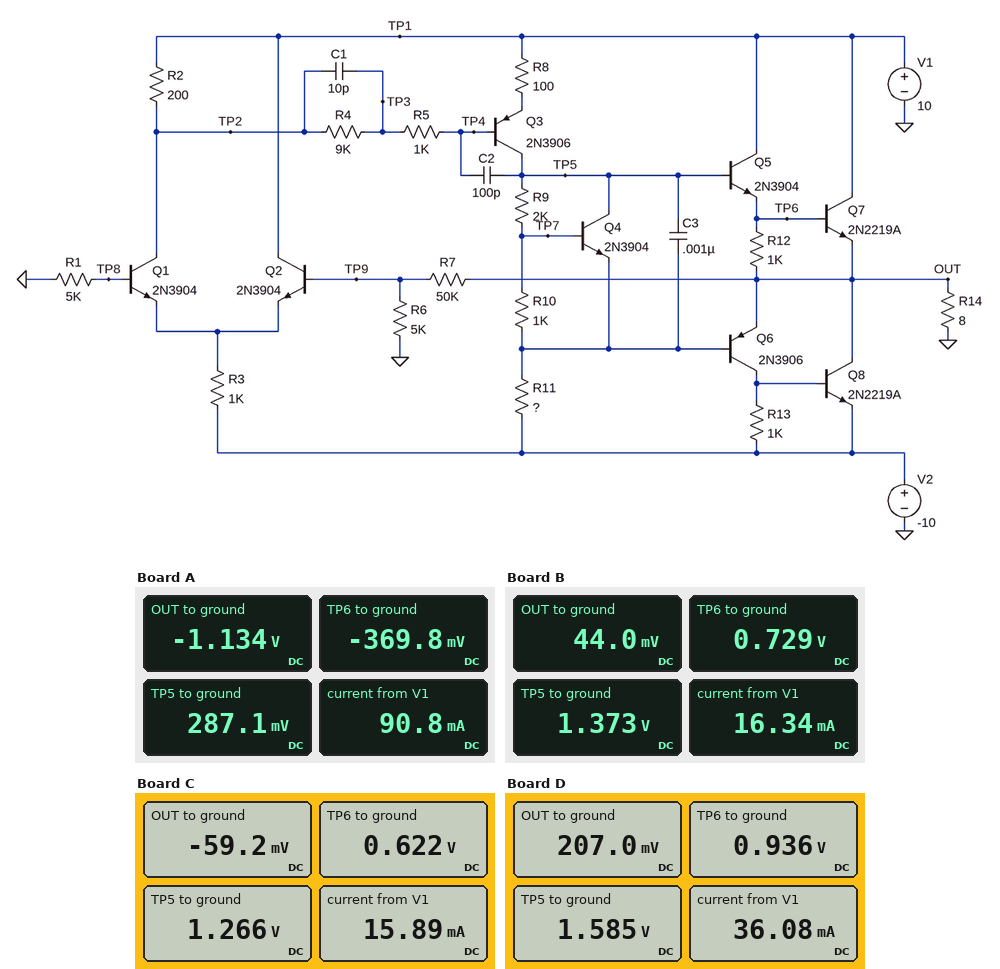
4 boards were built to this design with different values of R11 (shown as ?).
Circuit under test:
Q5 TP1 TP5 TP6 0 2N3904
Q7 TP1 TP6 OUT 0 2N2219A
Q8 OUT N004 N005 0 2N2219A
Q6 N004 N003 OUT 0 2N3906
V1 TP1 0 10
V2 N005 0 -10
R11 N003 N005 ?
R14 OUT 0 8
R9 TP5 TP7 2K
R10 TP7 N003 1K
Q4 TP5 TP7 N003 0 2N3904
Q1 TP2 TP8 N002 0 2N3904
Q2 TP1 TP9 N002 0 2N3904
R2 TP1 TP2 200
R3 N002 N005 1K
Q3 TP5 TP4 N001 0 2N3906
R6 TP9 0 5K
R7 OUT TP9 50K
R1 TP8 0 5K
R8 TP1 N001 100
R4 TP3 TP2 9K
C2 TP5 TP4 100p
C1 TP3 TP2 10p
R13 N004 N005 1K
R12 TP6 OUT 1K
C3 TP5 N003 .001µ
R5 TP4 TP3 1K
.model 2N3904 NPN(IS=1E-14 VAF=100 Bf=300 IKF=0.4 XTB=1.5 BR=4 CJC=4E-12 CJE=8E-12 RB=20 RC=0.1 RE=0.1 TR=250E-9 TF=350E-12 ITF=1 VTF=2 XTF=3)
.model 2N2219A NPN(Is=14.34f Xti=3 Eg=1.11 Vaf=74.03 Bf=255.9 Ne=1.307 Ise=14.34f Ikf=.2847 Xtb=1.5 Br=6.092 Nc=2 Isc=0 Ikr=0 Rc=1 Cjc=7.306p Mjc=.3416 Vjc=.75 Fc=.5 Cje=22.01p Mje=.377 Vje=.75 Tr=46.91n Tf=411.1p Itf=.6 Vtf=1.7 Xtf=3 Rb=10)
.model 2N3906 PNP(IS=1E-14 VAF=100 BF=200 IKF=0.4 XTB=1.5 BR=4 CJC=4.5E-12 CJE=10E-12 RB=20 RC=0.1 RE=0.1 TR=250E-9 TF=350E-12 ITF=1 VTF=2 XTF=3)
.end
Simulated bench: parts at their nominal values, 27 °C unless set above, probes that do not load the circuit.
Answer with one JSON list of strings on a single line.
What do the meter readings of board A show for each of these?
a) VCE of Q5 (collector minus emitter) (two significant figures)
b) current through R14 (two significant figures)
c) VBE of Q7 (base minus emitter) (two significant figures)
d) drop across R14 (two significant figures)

["10 V", "140 mA", "760 mV", "1.1 V"]
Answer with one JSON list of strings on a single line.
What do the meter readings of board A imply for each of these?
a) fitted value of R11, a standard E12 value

["1.8 kΩ"]
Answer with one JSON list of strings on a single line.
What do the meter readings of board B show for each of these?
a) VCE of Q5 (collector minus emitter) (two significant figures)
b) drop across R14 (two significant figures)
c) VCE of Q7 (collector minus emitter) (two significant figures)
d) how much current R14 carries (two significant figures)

["9.3 V", "44 mV", "10 V", "5.5 mA"]
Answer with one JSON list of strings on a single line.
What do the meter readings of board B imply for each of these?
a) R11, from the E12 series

["6.8 kΩ"]
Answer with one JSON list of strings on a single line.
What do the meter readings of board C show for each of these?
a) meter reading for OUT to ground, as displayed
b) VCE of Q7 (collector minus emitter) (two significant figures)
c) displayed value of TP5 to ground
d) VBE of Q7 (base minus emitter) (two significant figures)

["-59.2 mV", "10 V", "1.266 V", "680 mV"]
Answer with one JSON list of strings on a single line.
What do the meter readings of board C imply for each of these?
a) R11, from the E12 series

["5.6 kΩ"]
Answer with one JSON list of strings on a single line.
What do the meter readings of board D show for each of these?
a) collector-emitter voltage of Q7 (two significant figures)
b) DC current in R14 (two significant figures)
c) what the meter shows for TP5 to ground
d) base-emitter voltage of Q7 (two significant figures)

["9.8 V", "26 mA", "1.585 V", "730 mV"]
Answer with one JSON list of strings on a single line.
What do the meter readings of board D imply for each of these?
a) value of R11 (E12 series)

["10 kΩ"]
